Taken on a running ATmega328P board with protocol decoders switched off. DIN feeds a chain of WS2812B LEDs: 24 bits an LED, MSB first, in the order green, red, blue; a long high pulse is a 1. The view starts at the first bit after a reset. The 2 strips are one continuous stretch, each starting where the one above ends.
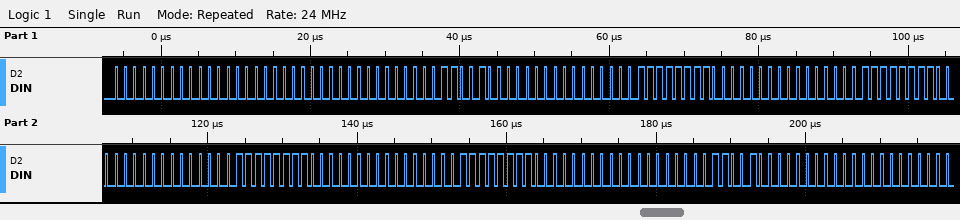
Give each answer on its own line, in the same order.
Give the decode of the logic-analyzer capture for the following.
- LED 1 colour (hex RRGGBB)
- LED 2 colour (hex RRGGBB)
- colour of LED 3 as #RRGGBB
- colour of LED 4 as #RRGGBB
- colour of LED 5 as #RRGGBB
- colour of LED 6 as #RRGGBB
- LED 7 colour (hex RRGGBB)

#000000
#190000
#FF0000
#FF0000
#FF0000
#FF0000
#190000
